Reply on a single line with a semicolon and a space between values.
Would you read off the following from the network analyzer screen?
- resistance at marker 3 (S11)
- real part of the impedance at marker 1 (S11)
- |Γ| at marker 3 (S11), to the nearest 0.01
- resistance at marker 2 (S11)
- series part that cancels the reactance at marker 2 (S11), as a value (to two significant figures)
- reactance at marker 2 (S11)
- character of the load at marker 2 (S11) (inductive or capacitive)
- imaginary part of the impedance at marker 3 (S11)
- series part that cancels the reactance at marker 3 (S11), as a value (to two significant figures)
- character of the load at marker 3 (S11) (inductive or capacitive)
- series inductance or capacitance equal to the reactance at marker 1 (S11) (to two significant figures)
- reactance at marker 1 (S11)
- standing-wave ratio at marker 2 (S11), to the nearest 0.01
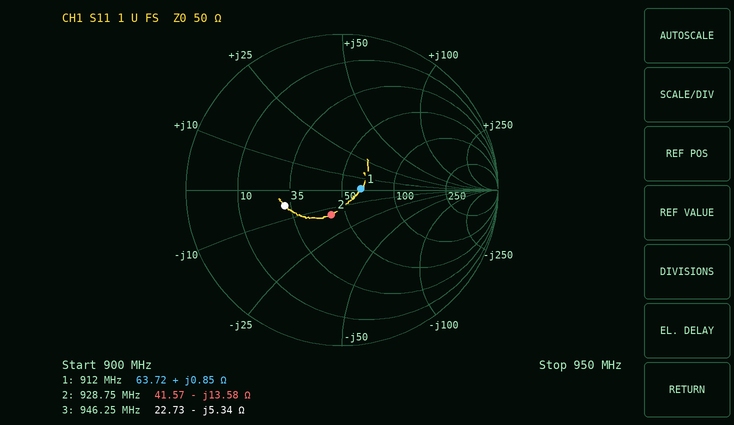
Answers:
22.73 Ω; 63.72 Ω; 0.38; 41.57 Ω; 2.3 nH; -13.58 Ω; capacitive; -5.34 Ω; 900 pH; capacitive; 150 pH; +0.85 Ω; 1.42
